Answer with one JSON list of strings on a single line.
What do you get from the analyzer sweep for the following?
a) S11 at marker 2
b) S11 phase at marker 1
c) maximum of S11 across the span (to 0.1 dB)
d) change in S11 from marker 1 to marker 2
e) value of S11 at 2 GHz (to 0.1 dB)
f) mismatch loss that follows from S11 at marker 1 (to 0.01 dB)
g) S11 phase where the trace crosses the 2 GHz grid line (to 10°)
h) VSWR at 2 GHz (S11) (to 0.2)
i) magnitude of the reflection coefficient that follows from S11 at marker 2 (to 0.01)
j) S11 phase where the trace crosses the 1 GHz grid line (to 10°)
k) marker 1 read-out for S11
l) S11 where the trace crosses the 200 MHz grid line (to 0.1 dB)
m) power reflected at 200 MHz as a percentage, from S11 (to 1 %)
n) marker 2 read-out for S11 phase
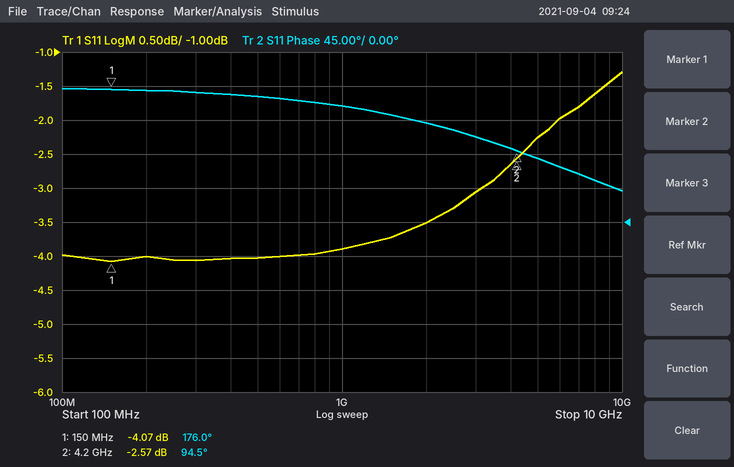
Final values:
["-2.57 dB", "176.0°", "-1.3 dB", "1.50 dB", "-3.5 dB", "2.16 dB", "130°", "5.0", "0.74", "150°", "-4.07 dB", "-4.0 dB", "40 %", "94.5°"]
